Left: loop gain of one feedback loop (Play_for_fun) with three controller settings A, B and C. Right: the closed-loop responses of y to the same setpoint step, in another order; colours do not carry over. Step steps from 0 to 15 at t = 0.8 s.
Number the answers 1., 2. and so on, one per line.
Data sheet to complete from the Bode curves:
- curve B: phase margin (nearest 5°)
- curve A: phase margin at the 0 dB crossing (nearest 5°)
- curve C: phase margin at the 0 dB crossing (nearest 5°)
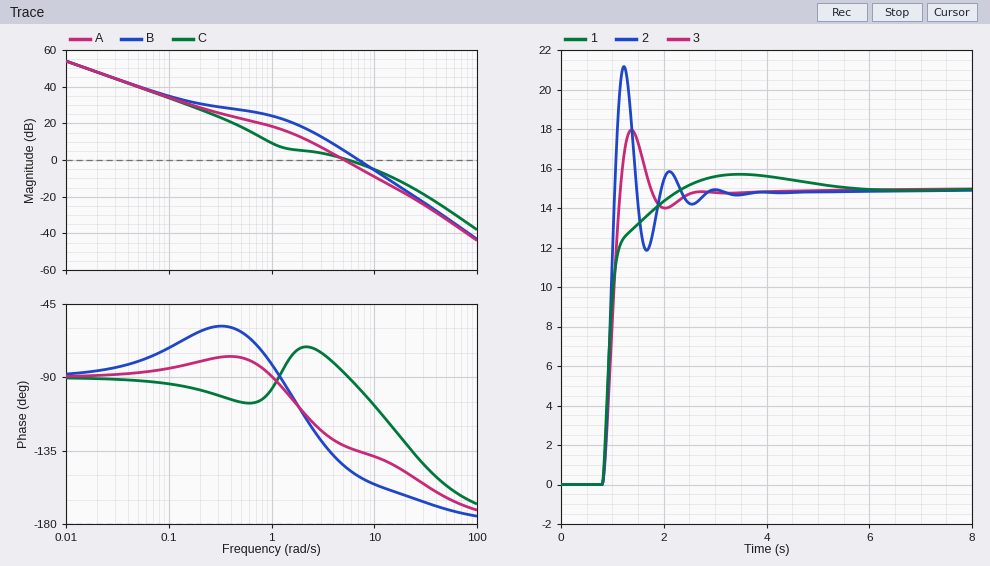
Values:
1. 30°
2. 50°
3. 90°
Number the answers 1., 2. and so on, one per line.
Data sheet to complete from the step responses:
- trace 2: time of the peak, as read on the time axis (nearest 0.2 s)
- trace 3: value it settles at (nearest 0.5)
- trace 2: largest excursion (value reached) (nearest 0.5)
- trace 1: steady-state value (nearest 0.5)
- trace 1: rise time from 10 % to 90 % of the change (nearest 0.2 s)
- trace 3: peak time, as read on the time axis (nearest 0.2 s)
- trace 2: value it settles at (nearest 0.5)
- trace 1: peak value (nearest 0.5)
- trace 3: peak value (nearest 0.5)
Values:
1. 1.2 s
2. 15.0
3. 21.0
4. 15.0
5. 0.8 s
6. 1.4 s
7. 15.0
8. 15.5
9. 18.0
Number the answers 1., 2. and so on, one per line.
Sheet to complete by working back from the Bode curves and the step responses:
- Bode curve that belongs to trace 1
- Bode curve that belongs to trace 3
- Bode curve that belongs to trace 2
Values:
1. C
2. A
3. B
